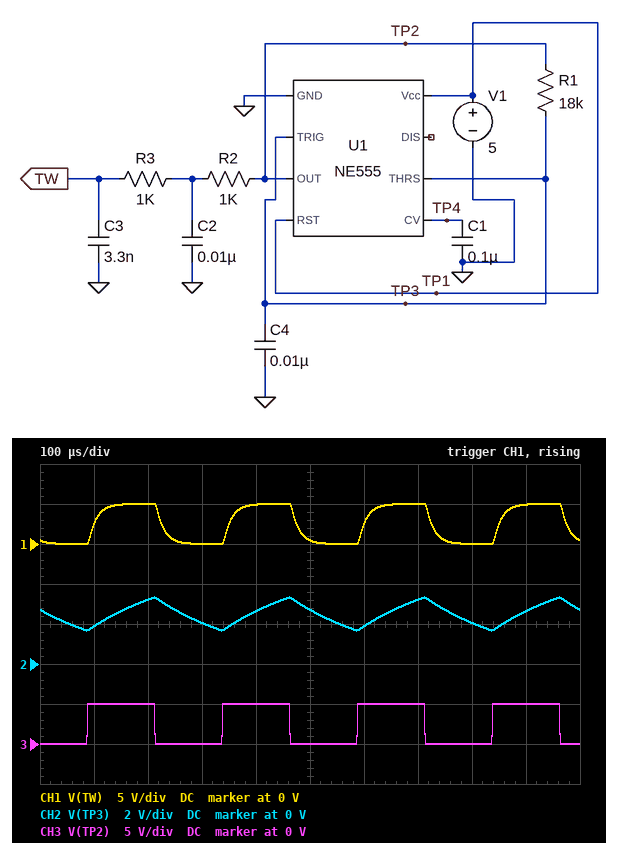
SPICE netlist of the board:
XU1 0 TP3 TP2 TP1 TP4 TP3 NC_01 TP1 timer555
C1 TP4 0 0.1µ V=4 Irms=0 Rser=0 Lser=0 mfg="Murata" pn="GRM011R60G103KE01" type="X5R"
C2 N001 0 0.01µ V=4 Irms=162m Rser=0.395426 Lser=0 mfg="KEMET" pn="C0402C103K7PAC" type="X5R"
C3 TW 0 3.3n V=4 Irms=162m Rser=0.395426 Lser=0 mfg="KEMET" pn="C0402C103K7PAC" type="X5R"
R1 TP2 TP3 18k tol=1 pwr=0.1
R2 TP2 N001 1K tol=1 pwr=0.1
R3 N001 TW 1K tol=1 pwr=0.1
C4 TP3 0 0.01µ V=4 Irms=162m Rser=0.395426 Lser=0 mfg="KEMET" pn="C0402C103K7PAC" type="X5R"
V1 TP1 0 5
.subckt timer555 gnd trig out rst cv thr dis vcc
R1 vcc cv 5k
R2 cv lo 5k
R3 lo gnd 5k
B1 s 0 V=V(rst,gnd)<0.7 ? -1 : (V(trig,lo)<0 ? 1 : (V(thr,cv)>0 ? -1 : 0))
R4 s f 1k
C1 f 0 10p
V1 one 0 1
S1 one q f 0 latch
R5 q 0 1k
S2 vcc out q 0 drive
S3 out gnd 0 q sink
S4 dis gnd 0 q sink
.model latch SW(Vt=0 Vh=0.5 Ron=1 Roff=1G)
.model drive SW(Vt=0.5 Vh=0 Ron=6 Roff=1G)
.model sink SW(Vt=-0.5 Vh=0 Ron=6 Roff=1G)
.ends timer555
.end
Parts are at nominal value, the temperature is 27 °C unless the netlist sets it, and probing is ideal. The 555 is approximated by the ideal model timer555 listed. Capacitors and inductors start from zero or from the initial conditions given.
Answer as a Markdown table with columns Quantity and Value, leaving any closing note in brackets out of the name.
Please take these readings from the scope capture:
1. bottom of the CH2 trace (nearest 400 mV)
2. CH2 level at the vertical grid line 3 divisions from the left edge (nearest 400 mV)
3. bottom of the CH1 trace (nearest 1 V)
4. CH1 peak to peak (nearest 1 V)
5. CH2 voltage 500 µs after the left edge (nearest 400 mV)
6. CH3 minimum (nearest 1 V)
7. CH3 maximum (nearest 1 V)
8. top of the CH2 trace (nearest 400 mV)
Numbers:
| Quantity | Value |
|---|---|
| bottom of the CH2 trace | 1.6 V |
| CH2 level at the vertical grid line 3 divisions from the left edge | 2.0 V |
| bottom of the CH1 trace | 0 V |
| CH1 peak to peak | 5 V |
| CH2 voltage 500 µs after the left edge | 2.8 V |
| CH3 minimum | 0 V |
| CH3 maximum | 5 V |
| top of the CH2 trace | 3.2 V |
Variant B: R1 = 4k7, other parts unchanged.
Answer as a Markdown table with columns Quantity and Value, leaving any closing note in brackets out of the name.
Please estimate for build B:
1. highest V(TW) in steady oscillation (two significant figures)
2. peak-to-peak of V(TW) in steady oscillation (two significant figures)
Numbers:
| Quantity | Value |
|---|---|
| highest V(TW) in steady oscillation | 4.4 V |
| peak-to-peak of V(TW) in steady oscillation | 3.9 V |
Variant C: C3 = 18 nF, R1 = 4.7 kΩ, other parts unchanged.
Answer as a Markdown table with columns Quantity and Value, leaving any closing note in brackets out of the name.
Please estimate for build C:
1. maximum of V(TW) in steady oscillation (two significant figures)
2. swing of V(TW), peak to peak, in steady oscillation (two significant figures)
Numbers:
| Quantity | Value |
|---|---|
| maximum of V(TW) in steady oscillation | 3.3 V |
| swing of V(TW), peak to peak, in steady oscillation | 1.6 V |
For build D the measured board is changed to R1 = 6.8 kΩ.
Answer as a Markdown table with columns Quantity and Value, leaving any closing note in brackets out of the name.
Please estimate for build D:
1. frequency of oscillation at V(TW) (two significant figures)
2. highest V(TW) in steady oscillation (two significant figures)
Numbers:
| Quantity | Value |
|---|---|
| frequency of oscillation at V(TW) | 11 kHz |
| highest V(TW) in steady oscillation | 4.8 V |
